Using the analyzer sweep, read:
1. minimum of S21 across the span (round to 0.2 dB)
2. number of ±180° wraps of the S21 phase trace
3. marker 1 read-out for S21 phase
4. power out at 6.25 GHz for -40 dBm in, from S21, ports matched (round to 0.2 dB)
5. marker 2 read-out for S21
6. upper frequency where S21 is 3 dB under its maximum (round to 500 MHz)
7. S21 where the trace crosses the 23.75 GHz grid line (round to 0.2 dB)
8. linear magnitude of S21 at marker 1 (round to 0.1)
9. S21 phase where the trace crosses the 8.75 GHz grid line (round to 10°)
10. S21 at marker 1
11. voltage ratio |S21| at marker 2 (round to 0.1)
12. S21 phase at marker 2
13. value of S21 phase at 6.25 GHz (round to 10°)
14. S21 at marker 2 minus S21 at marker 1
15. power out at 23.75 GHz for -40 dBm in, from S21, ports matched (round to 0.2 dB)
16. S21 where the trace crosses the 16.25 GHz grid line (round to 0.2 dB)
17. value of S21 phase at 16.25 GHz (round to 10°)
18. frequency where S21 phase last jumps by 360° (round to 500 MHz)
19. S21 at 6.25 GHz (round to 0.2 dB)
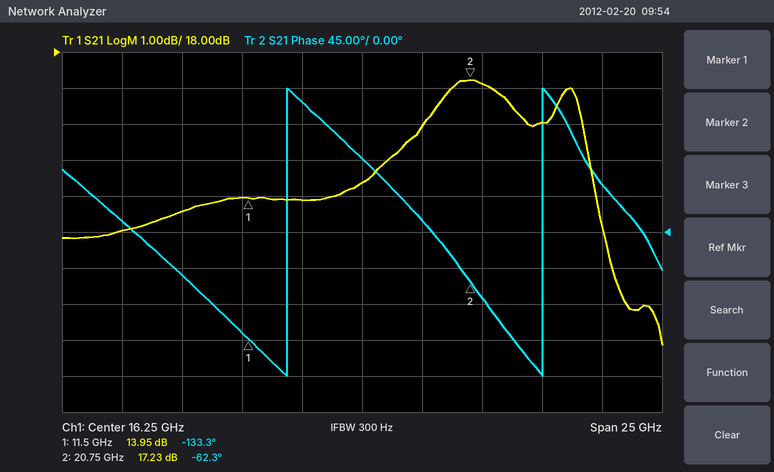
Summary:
9.8 dB
2
-133.3°
-27.0 dBm
17.23 dB
26.0 GHz
16.0 dB
5.0
-50°
13.95 dB
7.3
-62.3°
10°
3.28 dB
-24.0 dBm
14.4 dB
90°
24.0 GHz
13.0 dB
